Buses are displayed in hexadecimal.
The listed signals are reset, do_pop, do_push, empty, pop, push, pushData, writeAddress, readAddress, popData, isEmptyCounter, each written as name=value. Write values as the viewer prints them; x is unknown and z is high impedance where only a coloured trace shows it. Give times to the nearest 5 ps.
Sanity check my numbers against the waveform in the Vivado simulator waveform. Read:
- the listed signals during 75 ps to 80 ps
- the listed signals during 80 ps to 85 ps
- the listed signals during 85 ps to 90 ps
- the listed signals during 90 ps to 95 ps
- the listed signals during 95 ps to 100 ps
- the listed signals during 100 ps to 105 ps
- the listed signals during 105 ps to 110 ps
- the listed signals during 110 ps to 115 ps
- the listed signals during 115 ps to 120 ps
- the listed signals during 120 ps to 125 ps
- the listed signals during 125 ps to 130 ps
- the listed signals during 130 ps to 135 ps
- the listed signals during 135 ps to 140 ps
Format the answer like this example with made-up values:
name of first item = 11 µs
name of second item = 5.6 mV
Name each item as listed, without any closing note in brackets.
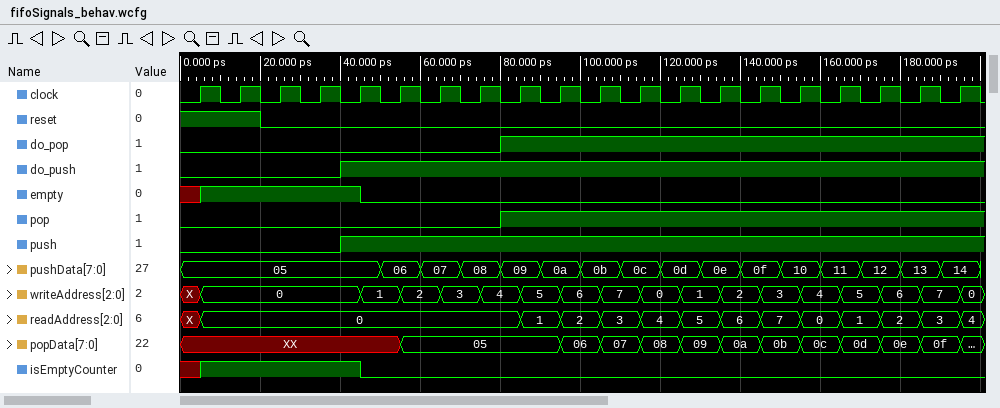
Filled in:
the listed signals during 75 ps to 80 ps = reset=0, do_pop=0, do_push=1, empty=0, pop=0, push=1, pushData=08, writeAddress=4, readAddress=0, popData=05, isEmptyCounter=0
the listed signals during 80 ps to 85 ps = reset=0, do_pop=1, do_push=1, empty=0, pop=1, push=1, pushData=09, writeAddress=4, readAddress=0, popData=05, isEmptyCounter=0
the listed signals during 85 ps to 90 ps = reset=0, do_pop=1, do_push=1, empty=0, pop=1, push=1, pushData=09, writeAddress=5, readAddress=1, popData=05, isEmptyCounter=0
the listed signals during 90 ps to 95 ps = reset=0, do_pop=1, do_push=1, empty=0, pop=1, push=1, pushData=0a, writeAddress=5, readAddress=1, popData=05, isEmptyCounter=0
the listed signals during 95 ps to 100 ps = reset=0, do_pop=1, do_push=1, empty=0, pop=1, push=1, pushData=0a, writeAddress=6, readAddress=2, popData=06, isEmptyCounter=0
the listed signals during 100 ps to 105 ps = reset=0, do_pop=1, do_push=1, empty=0, pop=1, push=1, pushData=0b, writeAddress=6, readAddress=2, popData=06, isEmptyCounter=0
the listed signals during 105 ps to 110 ps = reset=0, do_pop=1, do_push=1, empty=0, pop=1, push=1, pushData=0b, writeAddress=7, readAddress=3, popData=07, isEmptyCounter=0
the listed signals during 110 ps to 115 ps = reset=0, do_pop=1, do_push=1, empty=0, pop=1, push=1, pushData=0c, writeAddress=7, readAddress=3, popData=07, isEmptyCounter=0
the listed signals during 115 ps to 120 ps = reset=0, do_pop=1, do_push=1, empty=0, pop=1, push=1, pushData=0c, writeAddress=0, readAddress=4, popData=08, isEmptyCounter=0
the listed signals during 120 ps to 125 ps = reset=0, do_pop=1, do_push=1, empty=0, pop=1, push=1, pushData=0d, writeAddress=0, readAddress=4, popData=08, isEmptyCounter=0
the listed signals during 125 ps to 130 ps = reset=0, do_pop=1, do_push=1, empty=0, pop=1, push=1, pushData=0d, writeAddress=1, readAddress=5, popData=09, isEmptyCounter=0
the listed signals during 130 ps to 135 ps = reset=0, do_pop=1, do_push=1, empty=0, pop=1, push=1, pushData=0e, writeAddress=1, readAddress=5, popData=09, isEmptyCounter=0
the listed signals during 135 ps to 140 ps = reset=0, do_pop=1, do_push=1, empty=0, pop=1, push=1, pushData=0e, writeAddress=2, readAddress=6, popData=0a, isEmptyCounter=0
